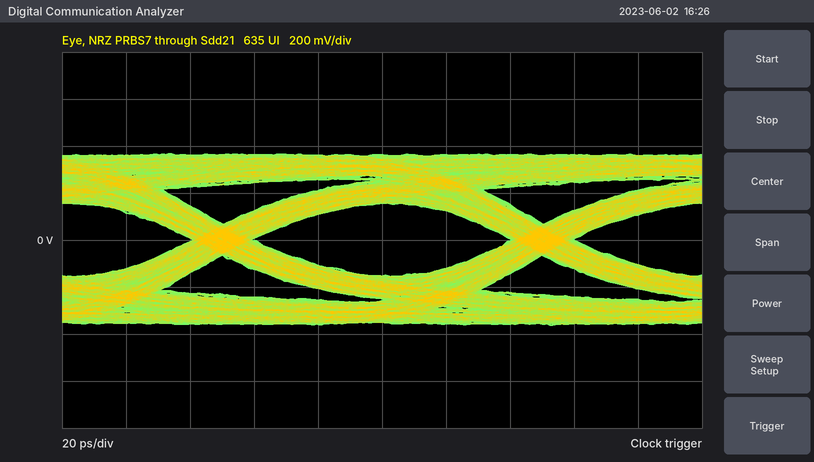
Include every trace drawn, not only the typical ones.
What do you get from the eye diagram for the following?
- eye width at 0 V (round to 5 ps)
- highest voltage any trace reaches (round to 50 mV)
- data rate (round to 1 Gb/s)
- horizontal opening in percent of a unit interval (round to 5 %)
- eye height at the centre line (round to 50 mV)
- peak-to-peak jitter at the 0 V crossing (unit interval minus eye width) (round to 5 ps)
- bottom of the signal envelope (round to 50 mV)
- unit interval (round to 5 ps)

80 ps
350 mV
10 Gb/s
80 %
300 mV
20 ps
-350 mV
100 ps
